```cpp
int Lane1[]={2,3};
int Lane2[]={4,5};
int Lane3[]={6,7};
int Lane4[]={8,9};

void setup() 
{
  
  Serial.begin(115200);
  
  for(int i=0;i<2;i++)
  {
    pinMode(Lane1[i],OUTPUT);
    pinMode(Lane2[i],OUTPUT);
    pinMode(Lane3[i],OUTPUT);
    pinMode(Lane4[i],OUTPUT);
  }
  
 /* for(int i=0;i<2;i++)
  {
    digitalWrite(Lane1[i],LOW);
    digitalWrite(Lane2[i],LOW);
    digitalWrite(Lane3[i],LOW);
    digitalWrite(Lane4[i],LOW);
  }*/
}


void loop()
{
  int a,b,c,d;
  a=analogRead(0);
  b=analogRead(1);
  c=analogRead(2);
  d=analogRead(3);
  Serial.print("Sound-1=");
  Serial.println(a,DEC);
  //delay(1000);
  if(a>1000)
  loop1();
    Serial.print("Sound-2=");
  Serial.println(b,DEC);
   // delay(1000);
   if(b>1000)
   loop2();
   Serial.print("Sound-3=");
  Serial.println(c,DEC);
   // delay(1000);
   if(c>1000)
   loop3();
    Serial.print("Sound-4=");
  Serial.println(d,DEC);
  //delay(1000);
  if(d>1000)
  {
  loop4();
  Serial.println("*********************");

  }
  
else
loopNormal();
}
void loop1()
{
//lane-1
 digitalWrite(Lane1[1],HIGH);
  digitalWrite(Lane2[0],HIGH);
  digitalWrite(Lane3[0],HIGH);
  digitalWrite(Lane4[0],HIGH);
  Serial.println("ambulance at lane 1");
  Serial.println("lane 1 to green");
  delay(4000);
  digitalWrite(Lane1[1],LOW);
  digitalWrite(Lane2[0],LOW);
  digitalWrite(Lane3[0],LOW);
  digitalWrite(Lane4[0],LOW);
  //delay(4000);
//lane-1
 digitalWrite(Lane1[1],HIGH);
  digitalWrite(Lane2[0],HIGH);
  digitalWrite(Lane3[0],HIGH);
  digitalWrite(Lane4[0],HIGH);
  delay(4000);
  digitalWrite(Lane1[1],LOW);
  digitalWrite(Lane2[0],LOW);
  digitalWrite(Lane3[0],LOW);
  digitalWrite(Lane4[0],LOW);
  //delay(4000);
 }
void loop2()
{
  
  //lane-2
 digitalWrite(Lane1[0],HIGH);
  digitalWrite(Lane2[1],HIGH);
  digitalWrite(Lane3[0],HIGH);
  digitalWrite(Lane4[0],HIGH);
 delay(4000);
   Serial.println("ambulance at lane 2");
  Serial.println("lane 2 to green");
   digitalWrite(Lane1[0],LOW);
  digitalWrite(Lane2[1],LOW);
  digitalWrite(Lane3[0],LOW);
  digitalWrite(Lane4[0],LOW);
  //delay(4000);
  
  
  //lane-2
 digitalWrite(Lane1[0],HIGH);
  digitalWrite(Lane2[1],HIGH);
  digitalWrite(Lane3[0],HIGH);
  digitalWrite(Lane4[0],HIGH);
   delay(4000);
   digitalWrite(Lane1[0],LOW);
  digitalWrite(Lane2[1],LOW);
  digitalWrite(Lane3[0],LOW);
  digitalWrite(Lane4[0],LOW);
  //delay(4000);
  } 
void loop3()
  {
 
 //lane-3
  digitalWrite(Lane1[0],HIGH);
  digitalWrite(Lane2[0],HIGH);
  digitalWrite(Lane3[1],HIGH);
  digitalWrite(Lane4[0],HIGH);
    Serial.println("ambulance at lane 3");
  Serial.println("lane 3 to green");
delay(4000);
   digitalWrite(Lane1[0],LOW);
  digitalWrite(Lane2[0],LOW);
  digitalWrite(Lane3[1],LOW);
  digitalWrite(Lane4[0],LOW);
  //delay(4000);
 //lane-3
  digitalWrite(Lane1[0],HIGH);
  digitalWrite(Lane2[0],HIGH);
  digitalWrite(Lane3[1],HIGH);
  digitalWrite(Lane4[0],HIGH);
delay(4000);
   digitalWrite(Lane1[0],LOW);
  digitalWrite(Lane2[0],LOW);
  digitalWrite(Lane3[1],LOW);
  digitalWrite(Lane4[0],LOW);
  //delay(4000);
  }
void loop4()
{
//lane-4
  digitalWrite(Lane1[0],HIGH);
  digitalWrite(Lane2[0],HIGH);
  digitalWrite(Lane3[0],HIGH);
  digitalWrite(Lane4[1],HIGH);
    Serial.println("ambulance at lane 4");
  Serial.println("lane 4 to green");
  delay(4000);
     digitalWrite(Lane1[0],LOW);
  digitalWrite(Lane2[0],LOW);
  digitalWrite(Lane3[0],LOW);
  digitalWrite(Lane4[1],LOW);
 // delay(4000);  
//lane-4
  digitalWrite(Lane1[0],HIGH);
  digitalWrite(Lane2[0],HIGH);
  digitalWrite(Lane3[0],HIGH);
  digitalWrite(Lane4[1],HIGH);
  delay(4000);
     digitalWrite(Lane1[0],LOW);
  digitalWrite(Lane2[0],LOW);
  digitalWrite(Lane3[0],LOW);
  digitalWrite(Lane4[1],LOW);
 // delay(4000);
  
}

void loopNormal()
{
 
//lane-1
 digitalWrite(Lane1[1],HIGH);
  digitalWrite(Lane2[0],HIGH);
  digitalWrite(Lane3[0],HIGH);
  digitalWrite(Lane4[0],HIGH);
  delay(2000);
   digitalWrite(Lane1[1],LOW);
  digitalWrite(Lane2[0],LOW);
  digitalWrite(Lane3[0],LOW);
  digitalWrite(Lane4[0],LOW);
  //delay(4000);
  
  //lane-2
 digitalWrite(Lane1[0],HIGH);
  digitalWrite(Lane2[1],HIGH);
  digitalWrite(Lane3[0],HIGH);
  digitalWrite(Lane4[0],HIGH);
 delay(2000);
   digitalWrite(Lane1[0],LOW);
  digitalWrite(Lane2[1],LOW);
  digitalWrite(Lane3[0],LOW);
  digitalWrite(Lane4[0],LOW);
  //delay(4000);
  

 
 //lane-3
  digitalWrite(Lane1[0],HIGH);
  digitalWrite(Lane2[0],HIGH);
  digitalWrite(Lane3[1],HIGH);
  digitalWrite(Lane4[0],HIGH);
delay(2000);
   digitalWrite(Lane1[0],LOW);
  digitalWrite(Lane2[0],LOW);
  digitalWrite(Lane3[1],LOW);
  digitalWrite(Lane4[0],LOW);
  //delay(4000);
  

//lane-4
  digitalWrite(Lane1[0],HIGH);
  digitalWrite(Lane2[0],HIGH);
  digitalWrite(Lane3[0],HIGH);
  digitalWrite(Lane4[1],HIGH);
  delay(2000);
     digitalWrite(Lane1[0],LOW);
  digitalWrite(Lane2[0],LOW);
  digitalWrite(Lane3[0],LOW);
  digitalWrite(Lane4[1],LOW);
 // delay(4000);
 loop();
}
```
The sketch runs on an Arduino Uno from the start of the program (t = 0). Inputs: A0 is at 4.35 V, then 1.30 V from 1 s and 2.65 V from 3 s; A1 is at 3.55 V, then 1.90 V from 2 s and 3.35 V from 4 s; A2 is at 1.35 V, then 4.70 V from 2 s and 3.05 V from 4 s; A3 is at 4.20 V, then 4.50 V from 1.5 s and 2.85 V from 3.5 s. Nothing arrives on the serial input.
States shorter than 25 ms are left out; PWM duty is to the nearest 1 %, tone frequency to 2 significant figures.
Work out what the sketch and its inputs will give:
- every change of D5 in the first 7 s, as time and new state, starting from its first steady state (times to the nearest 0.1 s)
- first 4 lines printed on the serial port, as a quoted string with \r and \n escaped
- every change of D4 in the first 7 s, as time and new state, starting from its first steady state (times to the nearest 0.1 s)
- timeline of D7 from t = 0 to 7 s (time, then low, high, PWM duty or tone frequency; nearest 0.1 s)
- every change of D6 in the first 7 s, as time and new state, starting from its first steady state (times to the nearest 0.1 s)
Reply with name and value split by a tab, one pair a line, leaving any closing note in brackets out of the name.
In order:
every change of D5 in the first 7 s, as time and new state, starting from its first steady state	0 s low; 2 s high; 4 s low
first 4 lines printed on the serial port, as a quoted string with \r and \n escaped	"Sound-1=890\r\nSound-2=727\r\nSound-3=276\r\nSound-4=860\r\n"
every change of D4 in the first 7 s, as time and new state, starting from its first steady state	0 s high; 2 s low; 4 s high
timeline of D7 from t = 0 to 7 s	0 s low; 4 s high; 6 s low
every change of D6 in the first 7 s, as time and new state, starting from its first steady state	0 s high; 4 s low; 6 s high
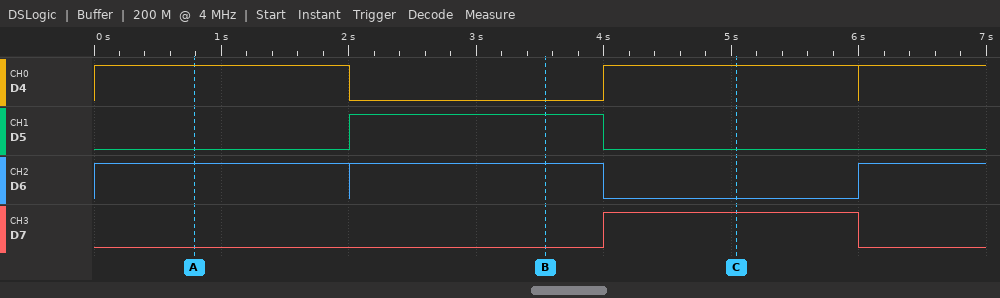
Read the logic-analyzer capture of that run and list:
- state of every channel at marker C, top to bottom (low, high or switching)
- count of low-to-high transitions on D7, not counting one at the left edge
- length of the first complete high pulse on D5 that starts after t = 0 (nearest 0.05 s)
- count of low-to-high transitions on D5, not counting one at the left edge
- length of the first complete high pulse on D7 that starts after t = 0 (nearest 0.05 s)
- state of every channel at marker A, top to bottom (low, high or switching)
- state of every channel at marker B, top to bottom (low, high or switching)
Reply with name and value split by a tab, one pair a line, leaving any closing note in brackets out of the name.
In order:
state of every channel at marker C, top to bottom	D4 high, D5 low, D6 low, D7 high
count of low-to-high transitions on D7, not counting one at the left edge	1
length of the first complete high pulse on D5 that starts after t = 0	2.00 s
count of low-to-high transitions on D5, not counting one at the left edge	1
length of the first complete high pulse on D7 that starts after t = 0	2.00 s
state of every channel at marker A, top to bottom	D4 high, D5 low, D6 high, D7 low
state of every channel at marker B, top to bottom	D4 low, D5 high, D6 high, D7 low
